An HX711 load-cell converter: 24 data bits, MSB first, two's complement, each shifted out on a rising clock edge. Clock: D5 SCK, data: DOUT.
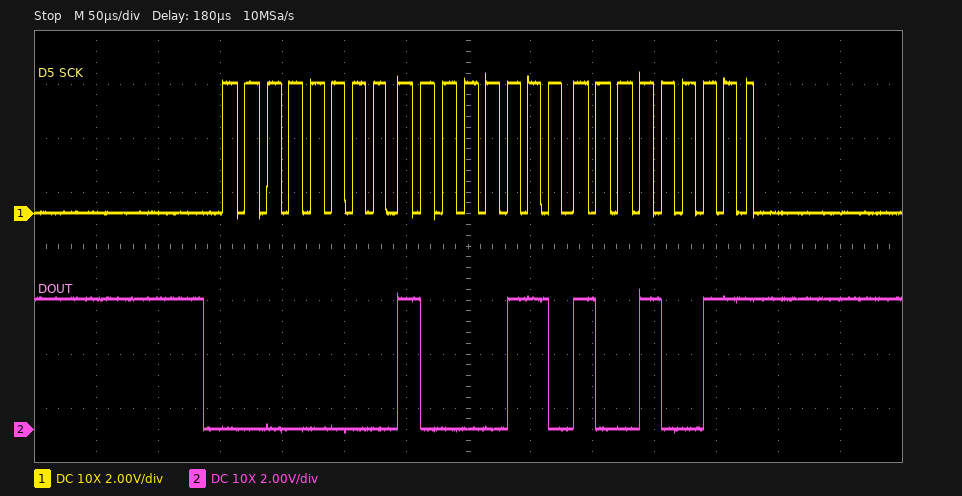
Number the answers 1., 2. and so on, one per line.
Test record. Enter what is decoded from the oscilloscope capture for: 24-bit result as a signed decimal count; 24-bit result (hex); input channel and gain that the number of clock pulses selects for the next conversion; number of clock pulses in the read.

1. 34451
2. 0x008693
3. channel A, gain 128
4. 25
